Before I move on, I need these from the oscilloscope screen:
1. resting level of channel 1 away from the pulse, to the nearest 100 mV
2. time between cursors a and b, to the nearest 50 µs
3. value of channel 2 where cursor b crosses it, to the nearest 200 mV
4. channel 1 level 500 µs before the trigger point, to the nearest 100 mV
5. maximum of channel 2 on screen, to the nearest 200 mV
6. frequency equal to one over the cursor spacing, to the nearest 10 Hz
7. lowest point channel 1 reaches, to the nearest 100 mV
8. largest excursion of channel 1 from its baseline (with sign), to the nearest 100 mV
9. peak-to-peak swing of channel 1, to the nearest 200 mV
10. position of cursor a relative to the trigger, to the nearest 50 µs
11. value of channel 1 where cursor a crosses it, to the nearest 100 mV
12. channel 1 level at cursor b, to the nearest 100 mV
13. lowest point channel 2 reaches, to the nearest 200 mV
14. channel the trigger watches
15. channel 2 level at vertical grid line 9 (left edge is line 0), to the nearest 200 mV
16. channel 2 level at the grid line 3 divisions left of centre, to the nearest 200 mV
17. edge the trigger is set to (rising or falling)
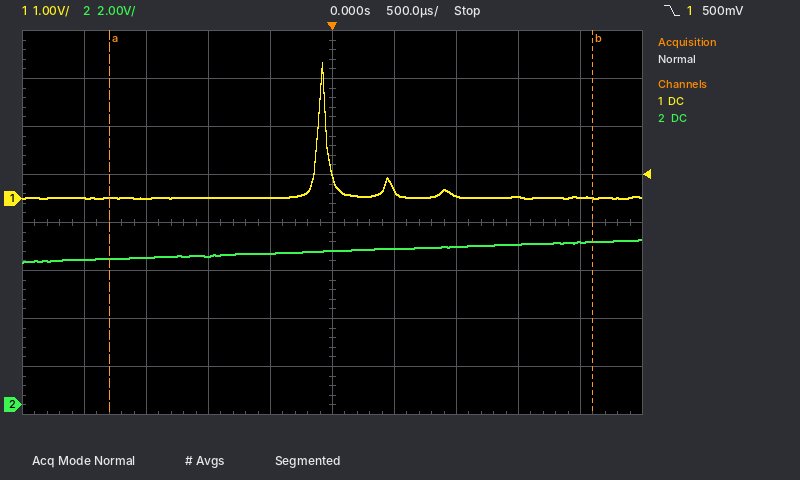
0.0 V
3.90 ms
6.8 V
0.0 V
6.8 V
260 Hz
0.0 V
+2.8 V
2.8 V
-1.80 ms
0.0 V
0.0 V
6.0 V
channel 1
6.8 V
6.2 V
falling
